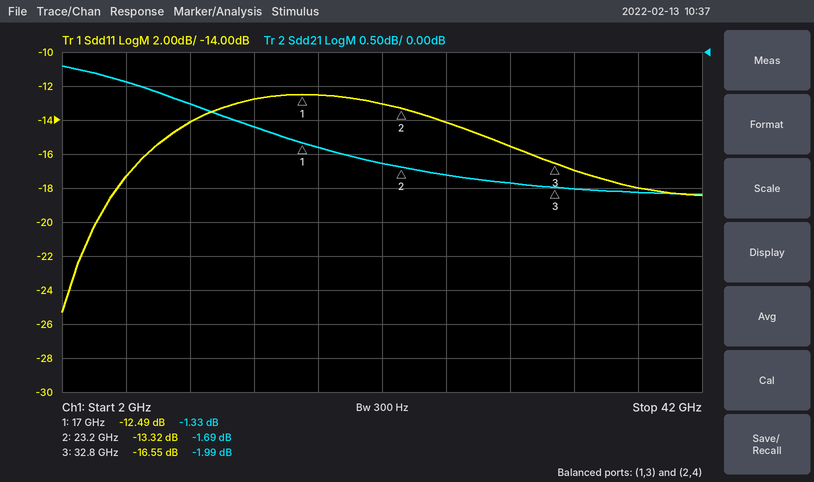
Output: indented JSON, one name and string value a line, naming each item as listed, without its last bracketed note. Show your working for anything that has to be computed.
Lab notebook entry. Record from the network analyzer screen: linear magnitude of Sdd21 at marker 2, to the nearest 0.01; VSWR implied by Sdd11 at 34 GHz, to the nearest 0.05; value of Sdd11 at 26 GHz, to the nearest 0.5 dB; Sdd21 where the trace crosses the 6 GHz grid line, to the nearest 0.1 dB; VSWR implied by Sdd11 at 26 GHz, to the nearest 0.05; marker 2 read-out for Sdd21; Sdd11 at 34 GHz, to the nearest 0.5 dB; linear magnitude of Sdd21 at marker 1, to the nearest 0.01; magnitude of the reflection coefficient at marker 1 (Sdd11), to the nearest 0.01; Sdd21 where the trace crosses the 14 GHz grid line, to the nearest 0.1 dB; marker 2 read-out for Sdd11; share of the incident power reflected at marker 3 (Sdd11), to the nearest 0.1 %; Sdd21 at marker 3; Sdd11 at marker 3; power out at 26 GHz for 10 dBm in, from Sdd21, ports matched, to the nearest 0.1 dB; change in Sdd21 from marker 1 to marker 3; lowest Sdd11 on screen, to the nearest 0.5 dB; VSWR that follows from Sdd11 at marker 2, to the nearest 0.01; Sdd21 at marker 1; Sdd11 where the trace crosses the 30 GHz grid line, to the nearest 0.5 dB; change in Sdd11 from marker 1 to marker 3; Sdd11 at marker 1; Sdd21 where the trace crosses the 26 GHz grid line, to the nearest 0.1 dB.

{
  "linear magnitude of Sdd21 at marker 2, to the nearest 0.01": "10^(-1.69/20) ≈ 0.82",
  "VSWR implied by Sdd11 at 34 GHz, to the nearest 0.05": "|Γ| = 10^(-17/20) = 0.1413; VSWR = (1 + 0.1413)/(1 − 0.1413) ≈ 1.33, so 1.35 to the nearest 0.05",
  "value of Sdd11 at 26 GHz, to the nearest 0.5 dB": "-14.0 dB",
  "Sdd21 where the trace crosses the 6 GHz grid line, to the nearest 0.1 dB": "-0.4 dB",
  "VSWR implied by Sdd11 at 26 GHz, to the nearest 0.05": "|Γ| = 10^(-14/20) = 0.1995; VSWR = (1 + 0.1995)/(1 − 0.1995) ≈ 1.50",
  "marker 2 read-out for Sdd21": "-1.69 dB",
  "Sdd11 at 34 GHz, to the nearest 0.5 dB": "-17.0 dB",
  "linear magnitude of Sdd21 at marker 1, to the nearest 0.01": "10^(-1.33/20) ≈ 0.86",
  "magnitude of the reflection coefficient at marker 1 (Sdd11), to the nearest 0.01": "10^(-12.49/20) ≈ 0.24",
  "Sdd21 where the trace crosses the 14 GHz grid line, to the nearest 0.1 dB": "-1.1 dB",
  "marker 2 read-out for Sdd11": "-13.32 dB",
  "share of the incident power reflected at marker 3 (Sdd11), to the nearest 0.1 %": "10^(-16.55/10) ≈ 2.2 %",
  "Sdd21 at marker 3": "-1.99 dB",
  "Sdd11 at marker 3": "-16.55 dB",
  "power out at 26 GHz for 10 dBm in, from Sdd21, ports matched, to the nearest 0.1 dB": "10 dBm + (-1.8 dB) = 8.2 dBm",
  "change in Sdd21 from marker 1 to marker 3": "-1.99 − (-1.33) = -0.66 dB",
  "lowest Sdd11 on screen, to the nearest 0.5 dB": "-25.5 dB",
  "VSWR that follows from Sdd11 at marker 2, to the nearest 0.01": "(1 + 0.2158)/(1 − 0.2158) ≈ 1.55",
  "Sdd21 at marker 1": "-1.33 dB",
  "Sdd11 where the trace crosses the 30 GHz grid line, to the nearest 0.5 dB": "-15.5 dB",
  "change in Sdd11 from marker 1 to marker 3": "-16.55 − (-12.49) = -4.06 dB",
  "Sdd11 at marker 1": "-12.49 dB",
  "Sdd21 where the trace crosses the 26 GHz grid line, to the nearest 0.1 dB": "-1.8 dB"
}
